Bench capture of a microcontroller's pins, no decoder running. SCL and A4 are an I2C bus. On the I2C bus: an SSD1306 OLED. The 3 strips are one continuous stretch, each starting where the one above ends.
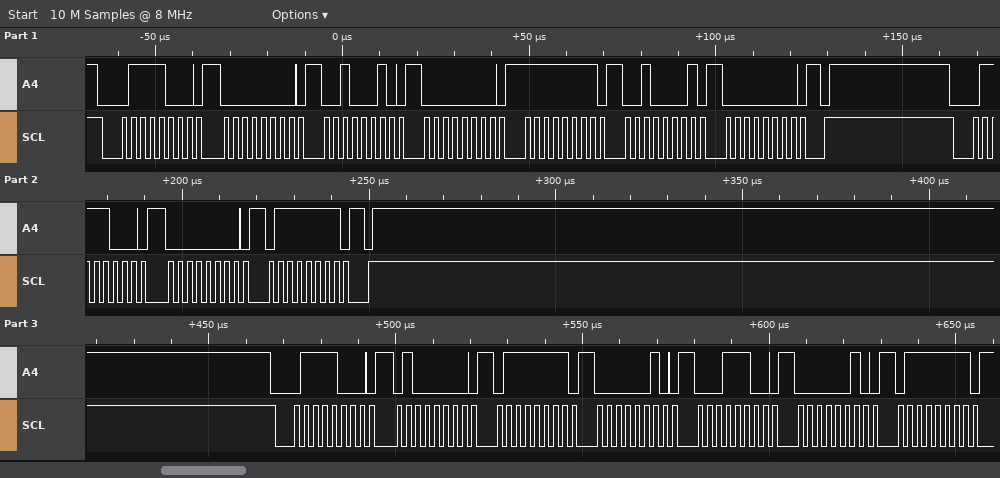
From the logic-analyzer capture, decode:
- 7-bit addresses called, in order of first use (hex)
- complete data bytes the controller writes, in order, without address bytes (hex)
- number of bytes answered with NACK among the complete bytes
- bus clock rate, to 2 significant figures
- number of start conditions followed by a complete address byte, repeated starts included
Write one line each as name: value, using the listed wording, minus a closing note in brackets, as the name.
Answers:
7-bit addresses called, in order of first use: 0x3C
complete data bytes the controller writes, in order, without address bytes: 00 22 00 FF 21 00 00 7F 40 7F 02 1C 02 7F
number of bytes answered with NACK among the complete bytes: 0
bus clock rate, to 2 significant figures: 400 kHz
number of start conditions followed by a complete address byte, repeated starts included: 3
